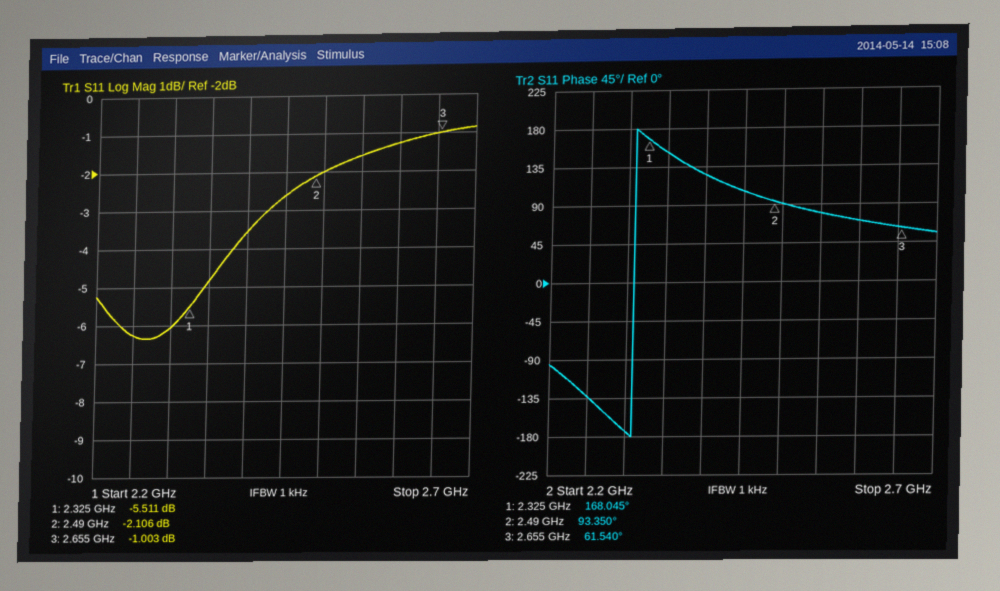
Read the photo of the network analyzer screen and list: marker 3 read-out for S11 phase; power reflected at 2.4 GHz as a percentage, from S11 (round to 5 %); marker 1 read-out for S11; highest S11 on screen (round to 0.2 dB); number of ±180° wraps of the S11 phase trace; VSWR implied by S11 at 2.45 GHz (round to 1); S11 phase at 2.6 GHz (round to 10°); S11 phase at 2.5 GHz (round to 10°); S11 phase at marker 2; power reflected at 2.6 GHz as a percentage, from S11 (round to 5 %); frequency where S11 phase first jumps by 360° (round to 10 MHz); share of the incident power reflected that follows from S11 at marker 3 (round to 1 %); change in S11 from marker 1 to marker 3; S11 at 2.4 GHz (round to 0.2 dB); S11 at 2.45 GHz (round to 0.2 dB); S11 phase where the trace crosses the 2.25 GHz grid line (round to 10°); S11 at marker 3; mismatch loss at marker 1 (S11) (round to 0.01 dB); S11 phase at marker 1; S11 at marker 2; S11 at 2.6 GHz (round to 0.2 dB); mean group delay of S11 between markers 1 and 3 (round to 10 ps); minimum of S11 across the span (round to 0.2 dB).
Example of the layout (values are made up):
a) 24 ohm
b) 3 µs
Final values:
a) 61.540°
b) 45 %
c) -5.511 dB
d) -0.8 dB
e) 1
f) 7
g) 70°
h) 90°
i) 93.350°
j) 75 %
k) 2.31 GHz
l) 79 %
m) 4.508 dB
n) -3.6 dB
o) -2.6 dB
p) -130°
q) -1.003 dB
r) 1.43 dB
s) 168.045°
t) -2.106 dB
u) -1.2 dB
v) 900 ps
w) -6.4 dB
